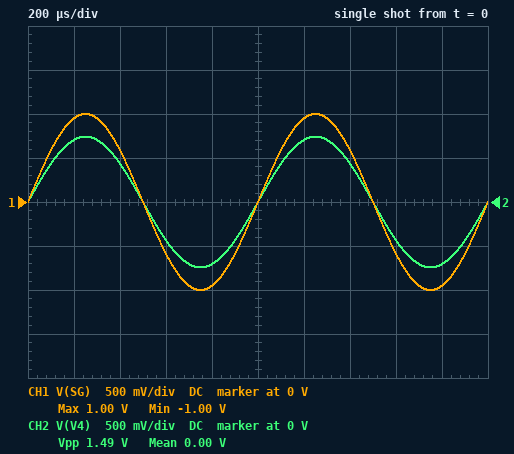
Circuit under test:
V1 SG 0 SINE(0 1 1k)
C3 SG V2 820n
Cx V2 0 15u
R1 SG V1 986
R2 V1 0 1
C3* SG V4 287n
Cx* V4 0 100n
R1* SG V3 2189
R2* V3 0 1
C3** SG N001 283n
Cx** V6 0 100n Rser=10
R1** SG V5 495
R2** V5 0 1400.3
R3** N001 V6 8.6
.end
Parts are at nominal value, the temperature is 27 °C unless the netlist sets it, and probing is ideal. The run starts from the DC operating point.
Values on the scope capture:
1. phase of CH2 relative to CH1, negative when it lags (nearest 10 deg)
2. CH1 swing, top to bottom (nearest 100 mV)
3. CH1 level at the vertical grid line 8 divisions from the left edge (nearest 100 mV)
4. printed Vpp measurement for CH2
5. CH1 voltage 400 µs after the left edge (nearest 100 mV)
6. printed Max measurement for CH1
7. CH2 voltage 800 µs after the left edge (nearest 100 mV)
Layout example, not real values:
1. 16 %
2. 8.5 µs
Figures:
1. 0 deg
2. 2.0 V
3. -600 mV
4. 1.49 V
5. 600 mV
6. 1.00 V
7. -700 mV
